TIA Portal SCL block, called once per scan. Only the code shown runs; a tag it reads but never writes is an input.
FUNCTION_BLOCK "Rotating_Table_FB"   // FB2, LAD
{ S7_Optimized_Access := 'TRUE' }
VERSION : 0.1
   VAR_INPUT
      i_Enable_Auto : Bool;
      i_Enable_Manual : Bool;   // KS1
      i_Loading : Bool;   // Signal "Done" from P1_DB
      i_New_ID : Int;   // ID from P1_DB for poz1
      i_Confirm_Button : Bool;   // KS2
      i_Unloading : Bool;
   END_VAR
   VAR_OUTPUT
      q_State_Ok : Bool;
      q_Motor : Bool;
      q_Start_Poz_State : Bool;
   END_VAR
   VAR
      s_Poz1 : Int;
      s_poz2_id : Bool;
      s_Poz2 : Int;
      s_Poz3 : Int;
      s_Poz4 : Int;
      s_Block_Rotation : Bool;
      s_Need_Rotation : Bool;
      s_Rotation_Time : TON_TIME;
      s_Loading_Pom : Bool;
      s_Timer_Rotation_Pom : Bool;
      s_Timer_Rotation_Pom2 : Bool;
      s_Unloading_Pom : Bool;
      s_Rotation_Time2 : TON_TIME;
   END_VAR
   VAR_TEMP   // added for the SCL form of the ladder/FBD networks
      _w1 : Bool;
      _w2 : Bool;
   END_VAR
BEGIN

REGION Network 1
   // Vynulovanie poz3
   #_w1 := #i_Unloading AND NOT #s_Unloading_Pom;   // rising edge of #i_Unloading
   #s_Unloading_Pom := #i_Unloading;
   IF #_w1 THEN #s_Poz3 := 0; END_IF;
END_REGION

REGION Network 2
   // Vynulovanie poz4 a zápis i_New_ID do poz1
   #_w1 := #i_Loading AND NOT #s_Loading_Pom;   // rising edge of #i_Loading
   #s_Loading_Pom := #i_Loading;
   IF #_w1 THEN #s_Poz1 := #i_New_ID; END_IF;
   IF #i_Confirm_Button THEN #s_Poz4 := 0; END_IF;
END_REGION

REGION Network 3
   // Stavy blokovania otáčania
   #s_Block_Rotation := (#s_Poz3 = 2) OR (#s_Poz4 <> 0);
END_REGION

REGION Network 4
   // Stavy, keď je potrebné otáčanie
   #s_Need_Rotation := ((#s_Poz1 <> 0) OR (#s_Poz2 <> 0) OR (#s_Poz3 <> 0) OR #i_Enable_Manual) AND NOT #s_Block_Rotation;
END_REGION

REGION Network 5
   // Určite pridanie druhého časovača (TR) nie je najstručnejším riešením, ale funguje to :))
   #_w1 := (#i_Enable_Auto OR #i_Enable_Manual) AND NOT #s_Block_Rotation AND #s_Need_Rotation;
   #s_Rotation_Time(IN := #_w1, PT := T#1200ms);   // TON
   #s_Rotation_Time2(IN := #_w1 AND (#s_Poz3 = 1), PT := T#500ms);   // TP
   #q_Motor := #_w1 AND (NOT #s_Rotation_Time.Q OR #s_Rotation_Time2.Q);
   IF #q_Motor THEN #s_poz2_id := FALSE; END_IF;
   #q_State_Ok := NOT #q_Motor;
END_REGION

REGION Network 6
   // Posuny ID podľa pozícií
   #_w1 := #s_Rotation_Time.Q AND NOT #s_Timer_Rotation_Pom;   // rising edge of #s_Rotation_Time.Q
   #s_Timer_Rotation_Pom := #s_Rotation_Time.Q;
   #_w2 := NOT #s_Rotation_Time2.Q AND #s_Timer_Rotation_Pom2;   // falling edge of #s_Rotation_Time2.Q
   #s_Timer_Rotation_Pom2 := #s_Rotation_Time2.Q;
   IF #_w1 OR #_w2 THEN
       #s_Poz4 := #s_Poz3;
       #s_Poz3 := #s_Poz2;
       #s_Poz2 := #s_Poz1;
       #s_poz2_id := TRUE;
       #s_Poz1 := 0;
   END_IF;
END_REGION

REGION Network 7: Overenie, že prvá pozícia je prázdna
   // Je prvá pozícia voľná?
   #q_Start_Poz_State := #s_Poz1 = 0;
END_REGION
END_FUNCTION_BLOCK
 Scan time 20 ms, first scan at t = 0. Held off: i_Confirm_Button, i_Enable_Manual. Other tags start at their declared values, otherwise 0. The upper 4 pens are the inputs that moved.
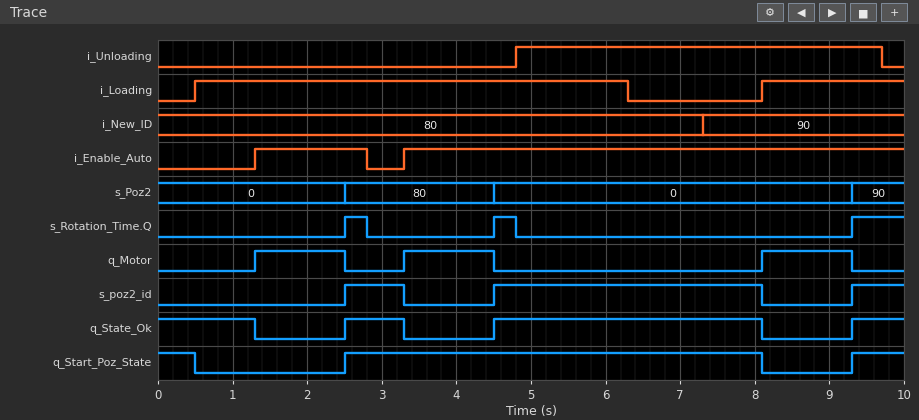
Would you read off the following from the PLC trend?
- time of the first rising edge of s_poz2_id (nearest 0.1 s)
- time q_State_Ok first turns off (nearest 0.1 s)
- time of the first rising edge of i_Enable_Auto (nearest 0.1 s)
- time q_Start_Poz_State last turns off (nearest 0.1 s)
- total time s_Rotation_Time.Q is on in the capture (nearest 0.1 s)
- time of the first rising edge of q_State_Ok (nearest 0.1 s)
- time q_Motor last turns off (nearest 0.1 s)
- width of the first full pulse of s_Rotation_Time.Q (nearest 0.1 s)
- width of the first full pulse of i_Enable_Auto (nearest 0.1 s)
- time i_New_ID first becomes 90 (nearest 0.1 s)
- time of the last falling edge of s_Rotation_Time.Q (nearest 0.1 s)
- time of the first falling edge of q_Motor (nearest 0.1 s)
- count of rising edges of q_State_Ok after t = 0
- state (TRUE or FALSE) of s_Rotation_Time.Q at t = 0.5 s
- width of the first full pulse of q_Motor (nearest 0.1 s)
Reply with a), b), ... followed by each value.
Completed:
a) 2.5 s
b) 1.3 s
c) 1.3 s
d) 8.1 s
e) 1.3 s
f) 2.5 s
g) 9.3 s
h) 0.3 s
i) 1.5 s
j) 7.3 s
k) 4.8 s
l) 2.5 s
m) 3
n) FALSE
o) 1.2 s
